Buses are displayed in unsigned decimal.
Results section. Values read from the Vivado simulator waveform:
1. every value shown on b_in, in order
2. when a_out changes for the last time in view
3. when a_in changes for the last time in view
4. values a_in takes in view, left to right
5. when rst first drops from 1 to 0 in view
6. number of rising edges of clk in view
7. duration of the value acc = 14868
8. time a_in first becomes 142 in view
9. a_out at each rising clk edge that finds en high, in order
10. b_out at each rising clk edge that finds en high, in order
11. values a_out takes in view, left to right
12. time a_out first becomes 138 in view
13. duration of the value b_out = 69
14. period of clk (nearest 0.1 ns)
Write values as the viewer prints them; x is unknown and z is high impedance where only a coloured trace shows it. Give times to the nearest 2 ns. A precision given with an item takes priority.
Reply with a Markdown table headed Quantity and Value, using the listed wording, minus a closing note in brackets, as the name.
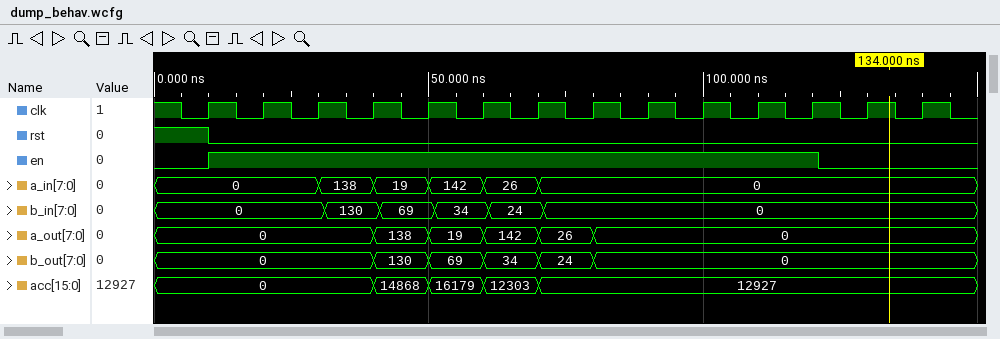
| Quantity | Value |
|---|---|
| every value shown on b_in, in order | 0, 130, 69, 34, 24, 0 |
| when a_out changes for the last time in view | 80 ns |
| when a_in changes for the last time in view | 70 ns |
| values a_in takes in view, left to right | 0, 138, 19, 142, 26, 0 |
| when rst first drops from 1 to 0 in view | 10 ns |
| number of rising edges of clk in view | 14 |
| duration of the value acc = 14868 | 10 ns |
| time a_in first becomes 142 in view | 50 ns |
| a_out at each rising clk edge that finds en high, in order | 0, 0, 0, 138, 19, 142, 26, 0, 0, 0, 0 |
| b_out at each rising clk edge that finds en high, in order | 0, 0, 0, 130, 69, 34, 24, 0, 0, 0, 0 |
| values a_out takes in view, left to right | 0, 138, 19, 142, 26, 0 |
| time a_out first becomes 138 in view | 40 ns |
| duration of the value b_out = 69 | 10 ns |
| period of clk | 10 ns |
